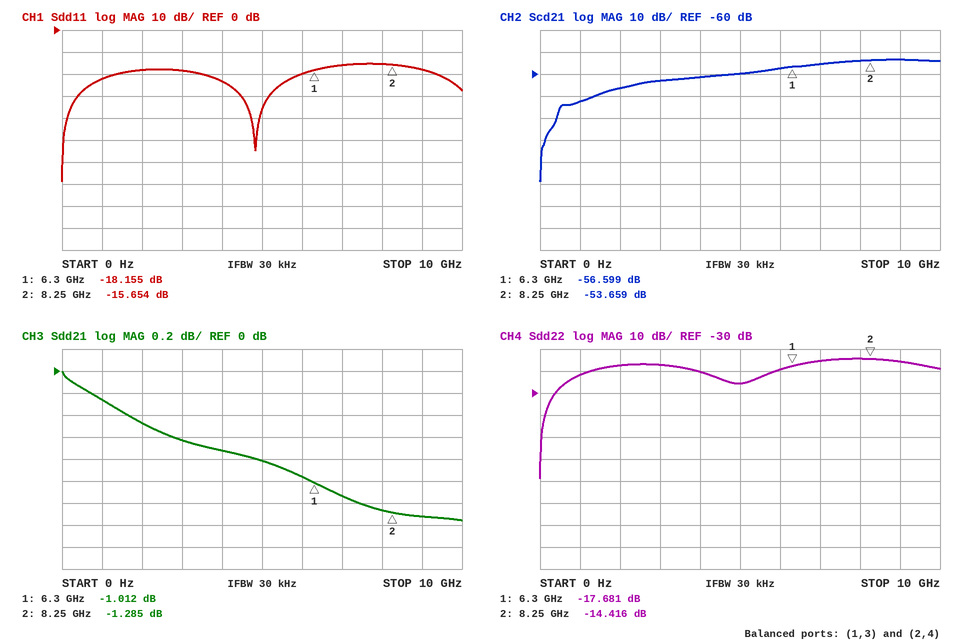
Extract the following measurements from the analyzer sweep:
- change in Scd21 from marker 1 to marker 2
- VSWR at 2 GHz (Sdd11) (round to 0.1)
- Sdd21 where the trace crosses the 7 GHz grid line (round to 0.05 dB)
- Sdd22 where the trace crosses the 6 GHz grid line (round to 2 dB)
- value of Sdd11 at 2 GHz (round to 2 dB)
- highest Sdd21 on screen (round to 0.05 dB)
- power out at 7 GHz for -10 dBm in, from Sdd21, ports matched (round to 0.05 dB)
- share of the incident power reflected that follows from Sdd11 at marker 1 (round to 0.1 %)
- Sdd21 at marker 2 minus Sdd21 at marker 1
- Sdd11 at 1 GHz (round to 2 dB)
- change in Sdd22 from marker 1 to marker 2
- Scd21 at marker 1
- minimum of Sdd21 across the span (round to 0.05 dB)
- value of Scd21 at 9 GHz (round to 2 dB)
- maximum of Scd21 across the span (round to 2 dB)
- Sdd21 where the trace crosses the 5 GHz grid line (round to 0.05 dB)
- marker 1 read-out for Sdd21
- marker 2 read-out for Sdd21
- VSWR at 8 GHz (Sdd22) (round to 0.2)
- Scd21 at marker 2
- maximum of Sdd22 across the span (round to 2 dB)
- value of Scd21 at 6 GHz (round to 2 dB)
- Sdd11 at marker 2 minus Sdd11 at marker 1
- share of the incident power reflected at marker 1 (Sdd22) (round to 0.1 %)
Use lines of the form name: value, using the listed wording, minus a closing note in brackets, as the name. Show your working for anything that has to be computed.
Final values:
change in Scd21 from marker 1 to marker 2: -53.659 − (-56.599) = 2.940 dB
VSWR at 2 GHz (Sdd11): |Γ| = 10^(-18/20) = 0.1259; VSWR = (1 + 0.1259)/(1 − 0.1259) ≈ 1.3
Sdd21 where the trace crosses the 7 GHz grid line: -1.15 dB
Sdd22 where the trace crosses the 6 GHz grid line: -20 dB
value of Sdd11 at 2 GHz: -18 dB
highest Sdd21 on screen: 0.00 dB
power out at 7 GHz for -10 dBm in, from Sdd21, ports matched: -10 dBm + (-1.15 dB) = -11.15 dBm
share of the incident power reflected that follows from Sdd11 at marker 1: 10^(-18.155/10) ≈ 1.5 %
Sdd21 at marker 2 minus Sdd21 at marker 1: -1.285 − (-1.012) = -0.273 dB
Sdd11 at 1 GHz: -22 dB
change in Sdd22 from marker 1 to marker 2: -14.416 − (-17.681) = 3.265 dB
Scd21 at marker 1: -56.599 dB
minimum of Sdd21 across the span: -1.35 dB
value of Scd21 at 9 GHz: -54 dB
maximum of Scd21 across the span: -54 dB
Sdd21 where the trace crosses the 5 GHz grid line: -0.80 dB
marker 1 read-out for Sdd21: -1.012 dB
marker 2 read-out for Sdd21: -1.285 dB
VSWR at 8 GHz (Sdd22): |Γ| = 10^(-14/20) = 0.1995; VSWR = (1 + 0.1995)/(1 − 0.1995) ≈ 1.50, so 1.4 to the nearest 0.2
Scd21 at marker 2: -53.659 dB
maximum of Sdd22 across the span: -14 dB
value of Scd21 at 6 GHz: -58 dB
Sdd11 at marker 2 minus Sdd11 at marker 1: -15.654 − (-18.155) = 2.501 dB
share of the incident power reflected at marker 1 (Sdd22): 10^(-17.681/10) ≈ 1.7 %
